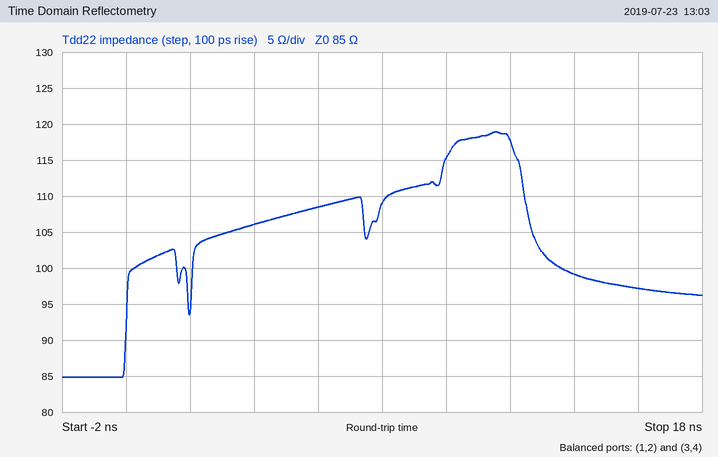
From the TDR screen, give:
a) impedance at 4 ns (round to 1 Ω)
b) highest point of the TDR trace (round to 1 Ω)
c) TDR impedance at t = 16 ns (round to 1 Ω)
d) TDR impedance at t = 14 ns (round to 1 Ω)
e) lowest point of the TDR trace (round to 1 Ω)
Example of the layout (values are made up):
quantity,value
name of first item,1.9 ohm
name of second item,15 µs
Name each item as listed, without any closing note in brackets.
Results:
quantity,value
impedance at 4 ns,106 Ω
highest point of the TDR trace,119 Ω
TDR impedance at t = 16 ns,97 Ω
TDR impedance at t = 14 ns,99 Ω
lowest point of the TDR trace,85 Ω
